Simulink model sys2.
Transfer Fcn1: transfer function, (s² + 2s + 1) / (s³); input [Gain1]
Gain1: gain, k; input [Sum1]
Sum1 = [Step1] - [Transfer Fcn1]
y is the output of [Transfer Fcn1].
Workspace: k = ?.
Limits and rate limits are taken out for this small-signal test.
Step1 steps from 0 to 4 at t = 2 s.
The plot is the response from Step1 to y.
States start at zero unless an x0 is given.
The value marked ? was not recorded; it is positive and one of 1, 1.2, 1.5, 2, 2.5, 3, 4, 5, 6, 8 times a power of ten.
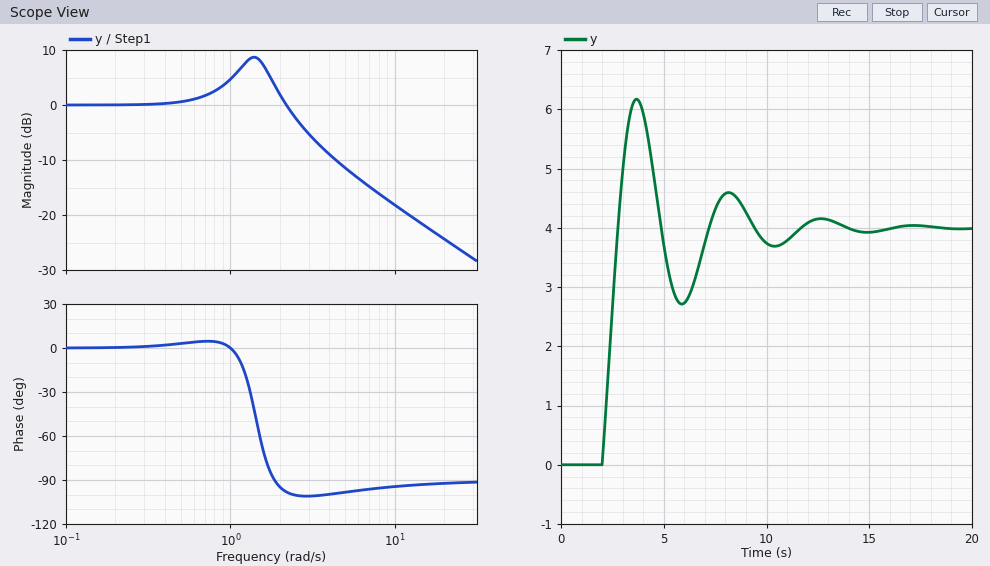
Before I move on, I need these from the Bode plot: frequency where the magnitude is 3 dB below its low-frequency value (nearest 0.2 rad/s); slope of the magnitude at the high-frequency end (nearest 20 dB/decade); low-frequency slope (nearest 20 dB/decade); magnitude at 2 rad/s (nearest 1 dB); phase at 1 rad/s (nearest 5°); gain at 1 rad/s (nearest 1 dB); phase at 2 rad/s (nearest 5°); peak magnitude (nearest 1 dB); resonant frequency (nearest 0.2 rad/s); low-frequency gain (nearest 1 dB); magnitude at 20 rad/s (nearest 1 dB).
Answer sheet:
2.6 rad/s
-20 dB/decade
0 dB/decade
2 dB
0°
5 dB
-95°
9 dB
1.4 rad/s
0 dB
-24 dB
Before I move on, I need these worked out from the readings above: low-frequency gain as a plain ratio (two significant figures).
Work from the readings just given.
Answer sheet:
1.0
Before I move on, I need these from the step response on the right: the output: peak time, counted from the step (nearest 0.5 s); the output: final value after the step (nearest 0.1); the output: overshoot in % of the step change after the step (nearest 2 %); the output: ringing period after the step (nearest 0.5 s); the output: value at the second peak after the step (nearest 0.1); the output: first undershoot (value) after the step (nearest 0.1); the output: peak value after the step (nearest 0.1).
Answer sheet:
1.5 s
4.0
54 %
4.5 s
4.6
2.7
6.2
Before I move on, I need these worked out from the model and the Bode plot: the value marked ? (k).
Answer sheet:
1.2
